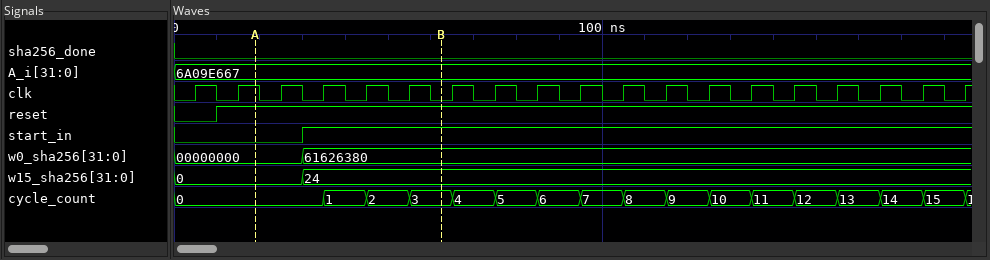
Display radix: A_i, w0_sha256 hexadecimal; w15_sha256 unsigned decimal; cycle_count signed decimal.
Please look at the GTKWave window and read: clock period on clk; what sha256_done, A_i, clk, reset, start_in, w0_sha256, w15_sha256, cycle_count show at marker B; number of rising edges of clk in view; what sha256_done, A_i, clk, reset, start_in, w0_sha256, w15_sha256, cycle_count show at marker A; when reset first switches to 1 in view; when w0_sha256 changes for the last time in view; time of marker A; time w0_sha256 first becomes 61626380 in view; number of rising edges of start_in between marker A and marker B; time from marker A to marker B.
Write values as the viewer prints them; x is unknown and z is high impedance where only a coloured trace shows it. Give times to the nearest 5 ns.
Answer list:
10 ns
sha256_done=0, A_i=6A09E667, clk=0, reset=1, start_in=1, w0_sha256=61626380, w15_sha256=24, cycle_count=3
19
sha256_done=0, A_i=6A09E667, clk=1, reset=1, start_in=0, w0_sha256=00000000, w15_sha256=0, cycle_count=0
10 ns
30 ns
20 ns
30 ns
1
45 ns
